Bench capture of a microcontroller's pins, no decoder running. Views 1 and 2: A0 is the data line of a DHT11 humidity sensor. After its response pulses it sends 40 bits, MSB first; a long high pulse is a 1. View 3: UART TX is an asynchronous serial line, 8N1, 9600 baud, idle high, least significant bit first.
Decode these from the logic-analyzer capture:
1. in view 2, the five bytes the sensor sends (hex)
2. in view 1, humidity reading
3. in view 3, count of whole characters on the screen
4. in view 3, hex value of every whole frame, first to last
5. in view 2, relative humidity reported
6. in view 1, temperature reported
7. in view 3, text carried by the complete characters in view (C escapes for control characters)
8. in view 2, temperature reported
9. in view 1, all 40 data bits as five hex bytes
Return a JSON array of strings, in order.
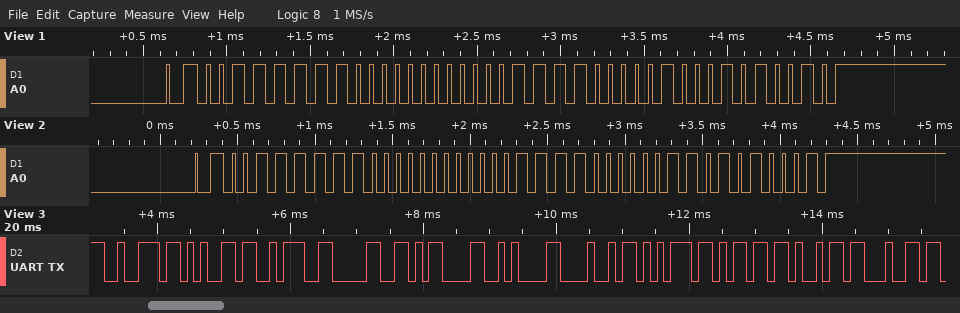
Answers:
["3F 00 0F 03 51", "63 %", "11", "72 65 3A 30 0D 0A 48 75 6D 69 64", "63 %", "15.4 °C", "\"re:0\\r\\nHumid\"", "15.3 °C", "3F 00 0F 04 52"]
